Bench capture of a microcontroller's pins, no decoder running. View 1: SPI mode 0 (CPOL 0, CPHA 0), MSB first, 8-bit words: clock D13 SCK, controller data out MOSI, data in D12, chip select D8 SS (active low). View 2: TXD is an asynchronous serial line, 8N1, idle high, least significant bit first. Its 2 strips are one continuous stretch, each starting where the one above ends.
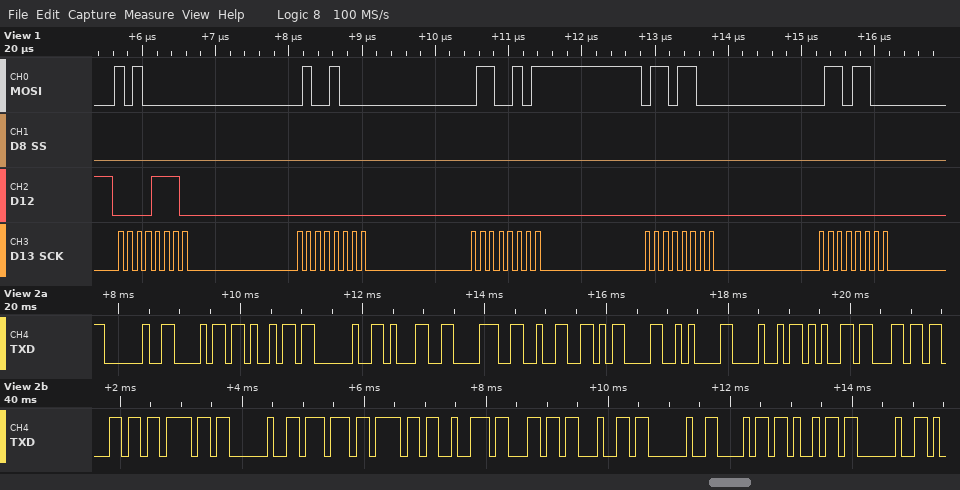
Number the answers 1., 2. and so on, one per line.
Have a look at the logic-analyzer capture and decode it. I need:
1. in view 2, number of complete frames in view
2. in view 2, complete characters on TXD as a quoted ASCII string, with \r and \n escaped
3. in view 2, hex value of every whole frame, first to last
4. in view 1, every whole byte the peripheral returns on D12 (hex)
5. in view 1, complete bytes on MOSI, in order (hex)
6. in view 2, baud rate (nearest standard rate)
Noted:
1. 24
2. " hi 182\r\nHello world hi "
3. 20 68 69 20 31 38 32 0D 0A 48 65 6C 6C 6F 20 77 6F 72 6C 64 20 68 69 20
4. 0x0E 0x00 0x00 0x00 0x00
5. 0xA0 0x48 0x65 0x6C 0x6C
6. 9600 baud
